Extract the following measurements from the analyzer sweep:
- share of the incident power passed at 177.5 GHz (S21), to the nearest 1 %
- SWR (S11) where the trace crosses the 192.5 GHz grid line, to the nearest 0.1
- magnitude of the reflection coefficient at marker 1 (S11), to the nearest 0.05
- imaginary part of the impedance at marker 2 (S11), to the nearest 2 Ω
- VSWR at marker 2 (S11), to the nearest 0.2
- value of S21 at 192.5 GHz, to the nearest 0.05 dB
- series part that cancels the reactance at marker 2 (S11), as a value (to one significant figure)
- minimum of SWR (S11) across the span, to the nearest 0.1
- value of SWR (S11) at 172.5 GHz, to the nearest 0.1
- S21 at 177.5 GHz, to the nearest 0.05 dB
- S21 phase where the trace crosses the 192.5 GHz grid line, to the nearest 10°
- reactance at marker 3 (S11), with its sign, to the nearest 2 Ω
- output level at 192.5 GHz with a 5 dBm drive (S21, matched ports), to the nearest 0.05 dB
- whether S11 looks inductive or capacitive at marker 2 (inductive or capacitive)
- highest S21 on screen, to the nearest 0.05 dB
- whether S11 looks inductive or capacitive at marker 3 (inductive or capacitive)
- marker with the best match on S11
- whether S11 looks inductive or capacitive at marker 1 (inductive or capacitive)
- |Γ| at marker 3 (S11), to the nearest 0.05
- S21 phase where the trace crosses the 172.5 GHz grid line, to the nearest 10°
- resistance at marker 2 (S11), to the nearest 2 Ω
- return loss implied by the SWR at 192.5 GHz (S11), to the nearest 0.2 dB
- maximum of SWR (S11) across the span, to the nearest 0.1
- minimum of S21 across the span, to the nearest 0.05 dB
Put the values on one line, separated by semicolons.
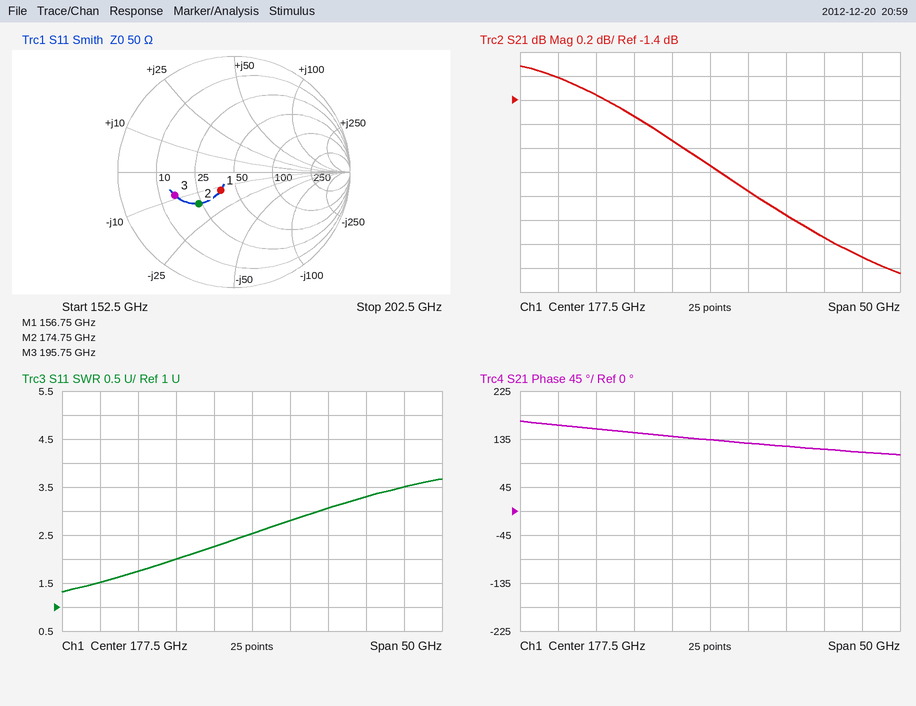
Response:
64 %; 3.3; 0.20; -16 Ω; 2.4; -2.55 dB; 10 pH; 1.3; 2.3; -1.95 dB; 120°; -8 Ω; 2.45 dBm; capacitive; -1.10 dB; capacitive; marker 1; capacitive; 0.55; 140°; 24 Ω; 5.4 dB; 3.7; -2.85 dB
